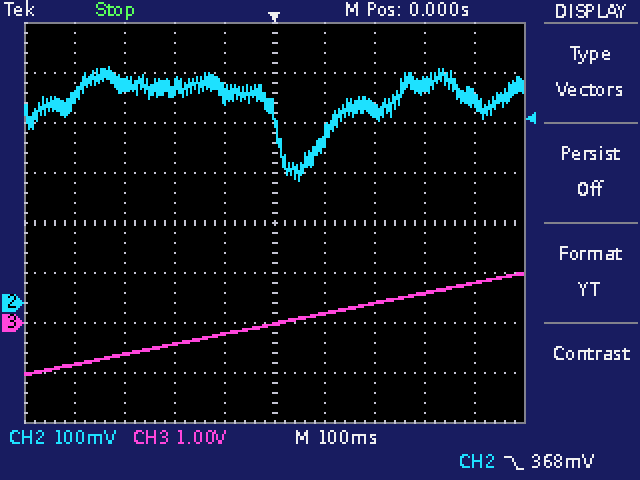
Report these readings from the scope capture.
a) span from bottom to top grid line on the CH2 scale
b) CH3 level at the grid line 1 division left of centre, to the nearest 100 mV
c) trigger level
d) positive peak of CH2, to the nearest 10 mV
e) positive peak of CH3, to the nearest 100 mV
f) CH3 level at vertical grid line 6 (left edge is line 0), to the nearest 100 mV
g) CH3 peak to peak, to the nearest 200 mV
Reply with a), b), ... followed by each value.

a) 800 mV
b) -200 mV
c) 368 mV
d) 470 mV
e) 1.0 V
f) 200 mV
g) 2.0 V
